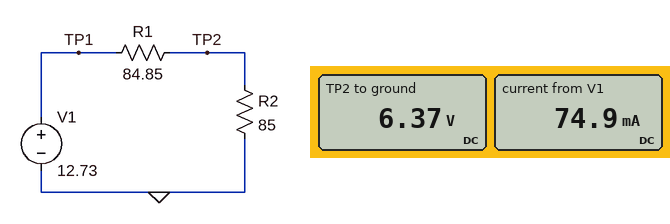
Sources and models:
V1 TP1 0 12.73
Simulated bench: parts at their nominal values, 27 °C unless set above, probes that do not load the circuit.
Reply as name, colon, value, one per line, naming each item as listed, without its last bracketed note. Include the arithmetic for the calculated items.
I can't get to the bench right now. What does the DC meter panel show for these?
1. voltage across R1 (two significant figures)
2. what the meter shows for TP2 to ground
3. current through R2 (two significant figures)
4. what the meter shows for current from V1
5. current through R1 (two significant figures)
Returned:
voltage across R1: 12.73 V - 6.37 V = 6.4 V
what the meter shows for TP2 to ground: 6.37 V
current through R2: (6.37 V) / 85 Ω = 75 mA
what the meter shows for current from V1: 74.9 mA
current through R1: (12.73 V - 6.37 V) / 84.85 Ω = 75 mA
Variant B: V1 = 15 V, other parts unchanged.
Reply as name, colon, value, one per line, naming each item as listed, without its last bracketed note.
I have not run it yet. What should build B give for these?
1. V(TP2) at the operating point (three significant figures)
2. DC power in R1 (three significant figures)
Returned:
V(TP2) at the operating point: 7.51 V
DC power in R1: 662 mW
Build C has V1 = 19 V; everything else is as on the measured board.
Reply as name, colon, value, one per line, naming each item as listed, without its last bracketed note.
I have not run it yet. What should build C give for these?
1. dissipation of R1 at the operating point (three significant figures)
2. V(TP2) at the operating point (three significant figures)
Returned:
dissipation of R1 at the operating point: 1.06 W
V(TP2) at the operating point: 9.51 V
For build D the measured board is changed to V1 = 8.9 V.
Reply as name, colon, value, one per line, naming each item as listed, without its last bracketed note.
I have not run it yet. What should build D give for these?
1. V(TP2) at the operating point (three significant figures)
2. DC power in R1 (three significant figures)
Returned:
V(TP2) at the operating point: 4.45 V
DC power in R1: 233 mW
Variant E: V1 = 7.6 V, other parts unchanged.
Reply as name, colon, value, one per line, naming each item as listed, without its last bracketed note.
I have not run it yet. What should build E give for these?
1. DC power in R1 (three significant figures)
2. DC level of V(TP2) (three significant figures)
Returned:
DC power in R1: 170 mW
DC level of V(TP2): 3.80 V
